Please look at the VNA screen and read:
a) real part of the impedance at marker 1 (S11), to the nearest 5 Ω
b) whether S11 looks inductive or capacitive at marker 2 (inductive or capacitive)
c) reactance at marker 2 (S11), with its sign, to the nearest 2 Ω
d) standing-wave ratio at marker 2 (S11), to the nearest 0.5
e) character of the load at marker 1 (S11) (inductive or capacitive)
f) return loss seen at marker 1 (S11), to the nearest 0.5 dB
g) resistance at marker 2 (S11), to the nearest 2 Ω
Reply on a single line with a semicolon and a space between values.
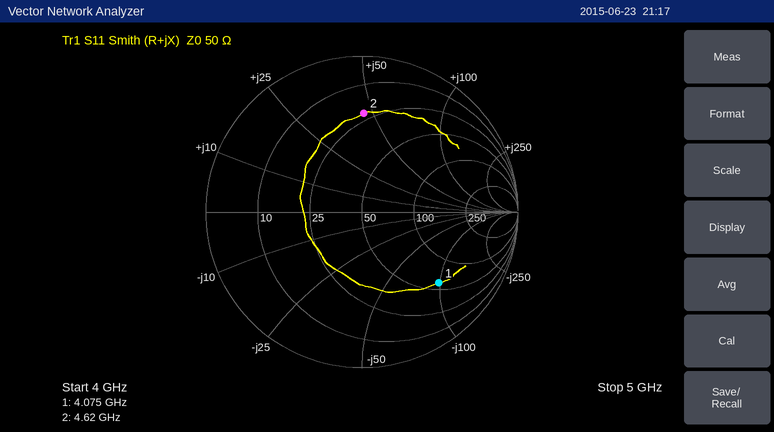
60 Ω; inductive; +46 Ω; 4.5; capacitive; 3.5 dB; 22 Ω
